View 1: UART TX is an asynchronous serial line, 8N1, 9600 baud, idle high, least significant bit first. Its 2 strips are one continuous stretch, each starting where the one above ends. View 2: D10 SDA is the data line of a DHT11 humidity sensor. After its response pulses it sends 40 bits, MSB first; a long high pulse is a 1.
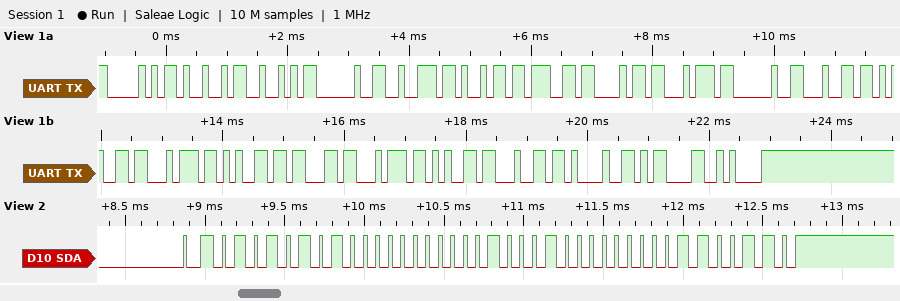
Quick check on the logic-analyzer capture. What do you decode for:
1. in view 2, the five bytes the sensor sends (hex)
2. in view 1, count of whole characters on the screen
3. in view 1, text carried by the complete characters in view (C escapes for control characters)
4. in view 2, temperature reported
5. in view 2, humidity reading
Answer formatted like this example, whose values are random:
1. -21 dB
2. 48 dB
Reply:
1. 55 00 11 00 66
2. 21
3. "PIR right detected!\r\n"
4. 17.0 °C
5. 85 %
